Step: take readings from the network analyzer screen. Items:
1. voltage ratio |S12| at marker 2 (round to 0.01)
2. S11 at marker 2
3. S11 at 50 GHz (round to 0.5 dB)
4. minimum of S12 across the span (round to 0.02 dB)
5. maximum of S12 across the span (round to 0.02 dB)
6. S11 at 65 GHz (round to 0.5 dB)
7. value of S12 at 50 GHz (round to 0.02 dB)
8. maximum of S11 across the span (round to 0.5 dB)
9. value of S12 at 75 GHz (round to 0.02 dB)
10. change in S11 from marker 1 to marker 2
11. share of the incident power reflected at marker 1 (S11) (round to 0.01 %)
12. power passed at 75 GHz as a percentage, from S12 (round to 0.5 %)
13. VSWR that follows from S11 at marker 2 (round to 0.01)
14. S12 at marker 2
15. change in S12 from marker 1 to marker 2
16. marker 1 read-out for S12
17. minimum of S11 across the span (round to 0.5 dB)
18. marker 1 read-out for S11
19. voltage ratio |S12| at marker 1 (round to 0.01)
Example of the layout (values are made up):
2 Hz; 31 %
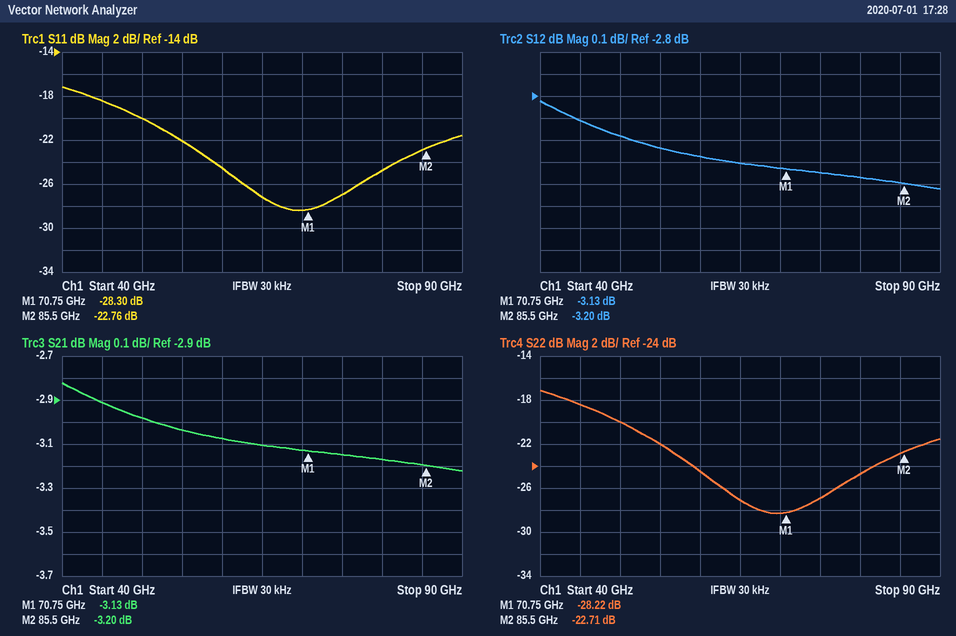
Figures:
0.69; -22.76 dB; -20.0 dB; -3.22 dB; -2.82 dB; -27.0 dB; -2.98 dB; -17.0 dB; -3.14 dB; 5.54 dB; 0.15 %; 48.5 %; 1.16; -3.20 dB; -0.07 dB; -3.13 dB; -28.5 dB; -28.30 dB; 0.70
